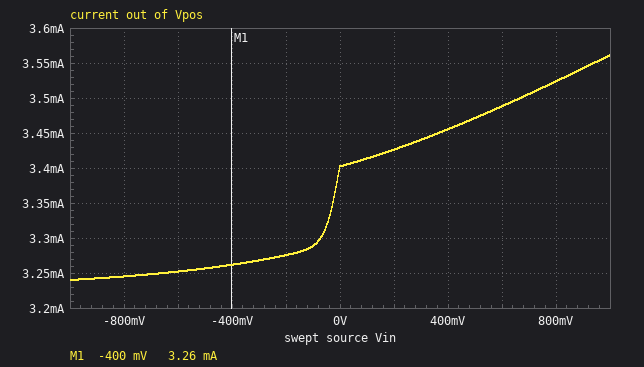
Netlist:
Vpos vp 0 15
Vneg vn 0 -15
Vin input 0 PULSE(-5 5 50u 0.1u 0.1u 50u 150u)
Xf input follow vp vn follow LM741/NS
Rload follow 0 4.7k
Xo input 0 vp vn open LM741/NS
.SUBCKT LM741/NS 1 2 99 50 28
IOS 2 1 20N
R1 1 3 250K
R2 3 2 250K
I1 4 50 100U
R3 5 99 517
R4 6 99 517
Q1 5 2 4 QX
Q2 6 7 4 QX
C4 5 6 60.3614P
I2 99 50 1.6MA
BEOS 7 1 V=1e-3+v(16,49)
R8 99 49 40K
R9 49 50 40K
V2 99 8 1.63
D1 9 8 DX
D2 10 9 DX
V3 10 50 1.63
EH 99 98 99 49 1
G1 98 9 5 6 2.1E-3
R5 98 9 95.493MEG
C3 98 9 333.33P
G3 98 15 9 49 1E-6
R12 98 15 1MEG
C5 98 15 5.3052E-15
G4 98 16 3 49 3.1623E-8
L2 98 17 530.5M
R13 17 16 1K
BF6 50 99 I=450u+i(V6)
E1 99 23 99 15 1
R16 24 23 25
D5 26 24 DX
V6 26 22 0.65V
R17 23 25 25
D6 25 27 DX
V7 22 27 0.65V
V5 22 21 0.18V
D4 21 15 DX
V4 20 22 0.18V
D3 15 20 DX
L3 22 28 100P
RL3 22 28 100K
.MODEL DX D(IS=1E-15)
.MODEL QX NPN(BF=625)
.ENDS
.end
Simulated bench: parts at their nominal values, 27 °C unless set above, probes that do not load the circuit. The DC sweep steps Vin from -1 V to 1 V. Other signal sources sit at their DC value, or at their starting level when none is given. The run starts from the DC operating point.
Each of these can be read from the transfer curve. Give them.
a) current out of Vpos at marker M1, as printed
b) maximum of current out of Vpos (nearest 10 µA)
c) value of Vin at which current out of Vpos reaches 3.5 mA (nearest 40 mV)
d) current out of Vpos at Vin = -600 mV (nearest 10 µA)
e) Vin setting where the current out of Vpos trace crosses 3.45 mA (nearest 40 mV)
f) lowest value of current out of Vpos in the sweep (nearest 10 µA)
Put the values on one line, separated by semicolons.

3.26 mA; 3.56 mA; 680 mV; 3.25 mA; 360 mV; 3.24 mA
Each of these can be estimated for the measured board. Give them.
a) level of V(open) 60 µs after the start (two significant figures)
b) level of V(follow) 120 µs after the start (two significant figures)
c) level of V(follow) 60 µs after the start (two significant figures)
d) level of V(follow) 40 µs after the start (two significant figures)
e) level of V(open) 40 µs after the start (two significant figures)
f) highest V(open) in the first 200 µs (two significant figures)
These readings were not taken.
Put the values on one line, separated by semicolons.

-11 V; -1.3 V; -1.8 V; -5.0 V; -14 V; 2.3 V
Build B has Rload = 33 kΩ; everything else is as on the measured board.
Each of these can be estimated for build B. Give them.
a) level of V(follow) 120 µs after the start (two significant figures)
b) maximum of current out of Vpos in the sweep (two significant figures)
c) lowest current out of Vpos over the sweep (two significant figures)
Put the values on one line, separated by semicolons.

-1.4 V; 3.4 mA; 3.3 mA
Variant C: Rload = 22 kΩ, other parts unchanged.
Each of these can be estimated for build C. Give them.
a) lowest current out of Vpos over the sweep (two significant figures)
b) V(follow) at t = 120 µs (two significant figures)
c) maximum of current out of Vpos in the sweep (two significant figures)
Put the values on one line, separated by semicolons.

3.3 mA; -1.4 V; 3.4 mA
